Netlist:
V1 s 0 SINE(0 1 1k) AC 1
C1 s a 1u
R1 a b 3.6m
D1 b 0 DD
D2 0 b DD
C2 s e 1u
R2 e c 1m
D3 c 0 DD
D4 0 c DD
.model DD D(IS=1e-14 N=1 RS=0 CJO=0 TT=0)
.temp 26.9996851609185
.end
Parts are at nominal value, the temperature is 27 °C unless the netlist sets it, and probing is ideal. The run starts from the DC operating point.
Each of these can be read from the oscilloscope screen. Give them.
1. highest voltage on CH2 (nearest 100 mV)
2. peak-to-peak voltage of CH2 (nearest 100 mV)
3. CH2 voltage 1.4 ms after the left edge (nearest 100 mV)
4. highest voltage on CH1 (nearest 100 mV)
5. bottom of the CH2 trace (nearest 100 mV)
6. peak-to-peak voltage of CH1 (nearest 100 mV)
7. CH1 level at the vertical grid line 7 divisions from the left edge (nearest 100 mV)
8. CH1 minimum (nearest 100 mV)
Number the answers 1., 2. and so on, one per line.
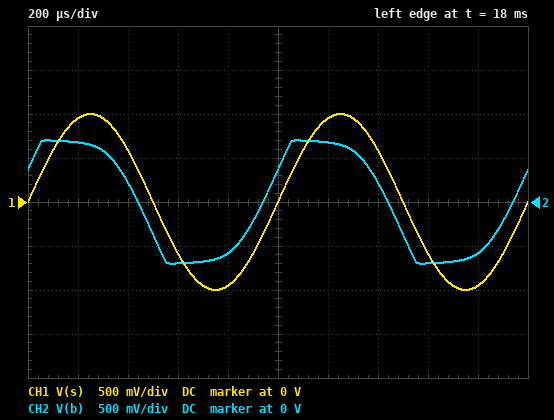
1. 700 mV
2. 1.4 V
3. 200 mV
4. 1.0 V
5. -700 mV
6. 2.0 V
7. 600 mV
8. -1.0 V
